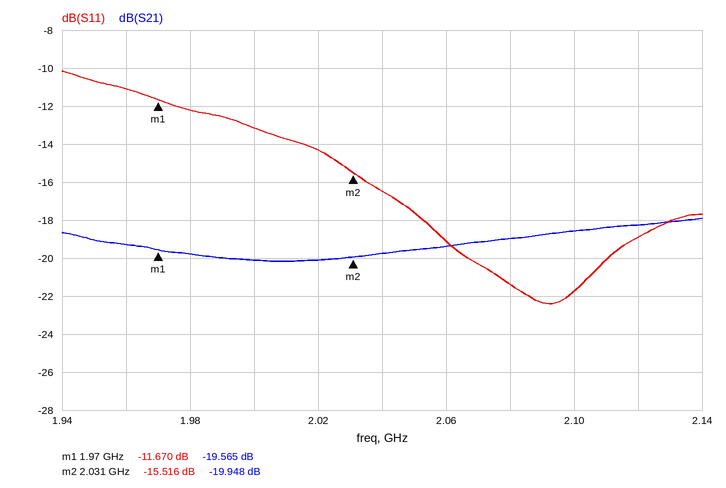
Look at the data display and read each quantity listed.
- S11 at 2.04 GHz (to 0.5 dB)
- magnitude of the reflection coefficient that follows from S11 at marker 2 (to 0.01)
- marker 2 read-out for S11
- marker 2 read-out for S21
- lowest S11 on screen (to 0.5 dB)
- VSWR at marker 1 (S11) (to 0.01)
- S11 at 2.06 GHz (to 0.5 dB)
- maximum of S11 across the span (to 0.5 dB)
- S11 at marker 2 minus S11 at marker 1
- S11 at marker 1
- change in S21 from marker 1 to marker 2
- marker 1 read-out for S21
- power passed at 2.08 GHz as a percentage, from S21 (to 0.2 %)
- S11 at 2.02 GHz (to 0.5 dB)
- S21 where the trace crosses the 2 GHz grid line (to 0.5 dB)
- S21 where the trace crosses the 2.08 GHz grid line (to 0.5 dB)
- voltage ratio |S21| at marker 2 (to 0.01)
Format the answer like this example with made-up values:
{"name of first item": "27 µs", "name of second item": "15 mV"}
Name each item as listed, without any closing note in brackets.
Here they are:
{"S11 at 2.04 GHz": "-16.5 dB", "magnitude of the reflection coefficient that follows from S11 at marker 2": "0.17", "marker 2 read-out for S11": "-15.516 dB", "marker 2 read-out for S21": "-19.948 dB", "lowest S11 on screen": "-22.5 dB", "VSWR at marker 1 (S11)": "1.71", "S11 at 2.06 GHz": "-19.0 dB", "maximum of S11 across the span": "-10.0 dB", "S11 at marker 2 minus S11 at marker 1": "-3.846 dB", "S11 at marker 1": "-11.670 dB", "change in S21 from marker 1 to marker 2": "-0.383 dB", "marker 1 read-out for S21": "-19.565 dB", "power passed at 2.08 GHz as a percentage, from S21": "1.2 %", "S11 at 2.02 GHz": "-14.5 dB", "S21 where the trace crosses the 2 GHz grid line": "-20.0 dB", "S21 where the trace crosses the 2.08 GHz grid line": "-19.0 dB", "voltage ratio |S21| at marker 2": "0.10"}
